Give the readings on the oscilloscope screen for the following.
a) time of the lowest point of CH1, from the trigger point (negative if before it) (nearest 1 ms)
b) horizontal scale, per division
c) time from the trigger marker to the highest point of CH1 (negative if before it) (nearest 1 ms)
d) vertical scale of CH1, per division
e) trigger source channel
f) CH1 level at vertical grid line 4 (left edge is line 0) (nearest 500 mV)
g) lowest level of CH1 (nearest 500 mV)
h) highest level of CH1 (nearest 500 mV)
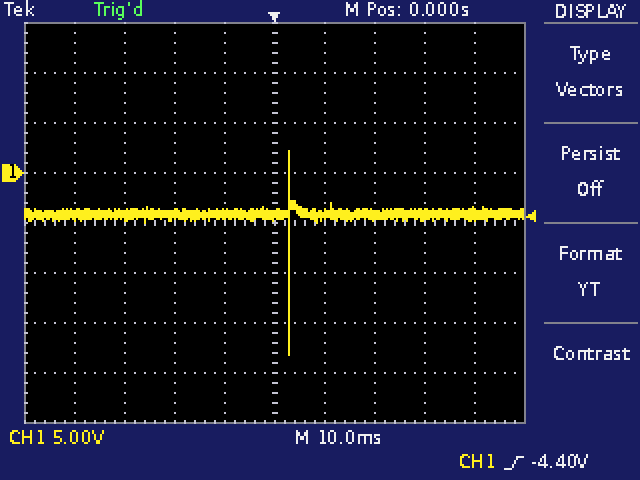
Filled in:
+3 ms
10 ms
+3 ms
5 V
CH1
-4.0 V
-18.0 V
2.0 V
